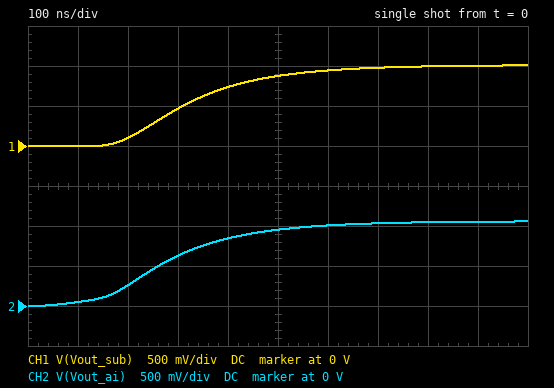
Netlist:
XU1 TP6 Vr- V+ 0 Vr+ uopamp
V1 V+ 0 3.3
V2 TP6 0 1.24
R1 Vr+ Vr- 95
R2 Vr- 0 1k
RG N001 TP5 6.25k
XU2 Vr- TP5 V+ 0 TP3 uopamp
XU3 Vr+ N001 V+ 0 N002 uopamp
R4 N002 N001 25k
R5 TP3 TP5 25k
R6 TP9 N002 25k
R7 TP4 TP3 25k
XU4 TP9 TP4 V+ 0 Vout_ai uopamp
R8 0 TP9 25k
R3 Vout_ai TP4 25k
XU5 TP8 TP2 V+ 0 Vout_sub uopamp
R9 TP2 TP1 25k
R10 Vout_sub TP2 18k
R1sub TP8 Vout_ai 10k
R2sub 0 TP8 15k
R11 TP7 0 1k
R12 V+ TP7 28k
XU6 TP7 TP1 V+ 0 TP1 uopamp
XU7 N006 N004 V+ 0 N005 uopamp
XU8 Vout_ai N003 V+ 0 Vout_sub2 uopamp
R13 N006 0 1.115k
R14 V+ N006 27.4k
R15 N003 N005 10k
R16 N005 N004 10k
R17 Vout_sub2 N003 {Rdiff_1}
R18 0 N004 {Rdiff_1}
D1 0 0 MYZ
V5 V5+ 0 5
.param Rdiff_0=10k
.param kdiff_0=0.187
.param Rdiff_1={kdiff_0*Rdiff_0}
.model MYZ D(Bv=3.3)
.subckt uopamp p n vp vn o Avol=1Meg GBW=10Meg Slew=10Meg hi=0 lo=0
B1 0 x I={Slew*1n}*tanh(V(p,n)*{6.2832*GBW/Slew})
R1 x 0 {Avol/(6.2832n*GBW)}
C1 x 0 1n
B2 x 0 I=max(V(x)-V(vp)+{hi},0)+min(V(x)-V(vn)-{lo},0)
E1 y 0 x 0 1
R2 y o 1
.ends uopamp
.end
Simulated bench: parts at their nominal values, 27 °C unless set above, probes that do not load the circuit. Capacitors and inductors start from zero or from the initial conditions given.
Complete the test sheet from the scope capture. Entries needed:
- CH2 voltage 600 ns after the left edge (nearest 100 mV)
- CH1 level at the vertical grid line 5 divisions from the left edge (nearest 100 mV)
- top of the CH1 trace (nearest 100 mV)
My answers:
1.0 V
900 mV
1.0 V
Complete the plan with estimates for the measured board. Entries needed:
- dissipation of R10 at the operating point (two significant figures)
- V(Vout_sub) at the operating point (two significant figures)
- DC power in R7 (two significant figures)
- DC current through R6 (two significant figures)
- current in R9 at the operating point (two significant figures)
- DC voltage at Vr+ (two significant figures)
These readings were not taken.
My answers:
7.9 µW
1.0 V
850 nW
37 µA
21 µA
1.4 V
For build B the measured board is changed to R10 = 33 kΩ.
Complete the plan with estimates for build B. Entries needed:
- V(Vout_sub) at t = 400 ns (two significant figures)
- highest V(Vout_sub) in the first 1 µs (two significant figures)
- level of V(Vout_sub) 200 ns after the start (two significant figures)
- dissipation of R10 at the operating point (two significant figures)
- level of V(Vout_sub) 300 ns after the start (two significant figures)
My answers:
920 mV
1.3 V
84 mV
14 µW
540 mV
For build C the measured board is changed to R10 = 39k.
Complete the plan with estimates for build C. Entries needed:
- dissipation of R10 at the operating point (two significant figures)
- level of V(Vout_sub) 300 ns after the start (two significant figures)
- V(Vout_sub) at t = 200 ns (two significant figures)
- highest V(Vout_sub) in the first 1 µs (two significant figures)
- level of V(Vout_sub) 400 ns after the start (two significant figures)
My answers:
17 µW
560 mV
79 mV
1.4 V
980 mV
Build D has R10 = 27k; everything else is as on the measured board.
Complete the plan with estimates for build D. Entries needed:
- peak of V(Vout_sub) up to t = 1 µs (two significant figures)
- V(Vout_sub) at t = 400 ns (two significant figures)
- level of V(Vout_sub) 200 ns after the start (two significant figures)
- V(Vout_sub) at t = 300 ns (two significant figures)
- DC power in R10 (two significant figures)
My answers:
1.2 V
850 mV
91 mV
510 mV
12 µW
